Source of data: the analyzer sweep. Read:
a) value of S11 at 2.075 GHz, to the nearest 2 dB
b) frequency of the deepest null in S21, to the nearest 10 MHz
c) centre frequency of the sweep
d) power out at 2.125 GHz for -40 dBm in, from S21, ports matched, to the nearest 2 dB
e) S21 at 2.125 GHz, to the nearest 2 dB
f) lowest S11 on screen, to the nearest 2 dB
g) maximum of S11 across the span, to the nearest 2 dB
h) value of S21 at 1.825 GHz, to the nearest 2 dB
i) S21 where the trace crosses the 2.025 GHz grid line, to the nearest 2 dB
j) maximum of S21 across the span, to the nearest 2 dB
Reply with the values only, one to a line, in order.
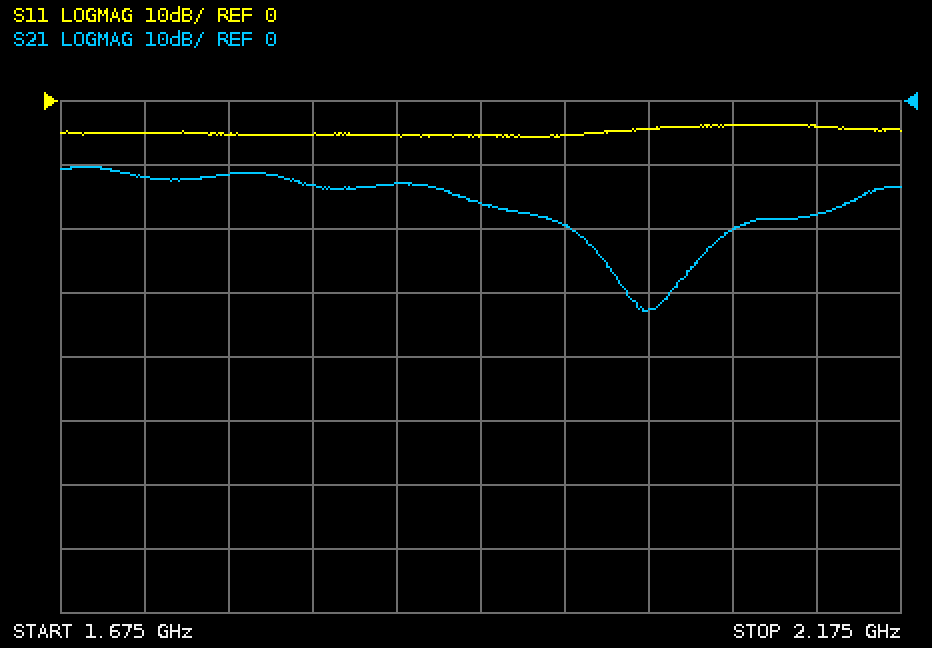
-4 dB
2.02 GHz
1.925 GHz
-58 dBm
-18 dB
-6 dB
-4 dB
-14 dB
-32 dB
-10 dB
